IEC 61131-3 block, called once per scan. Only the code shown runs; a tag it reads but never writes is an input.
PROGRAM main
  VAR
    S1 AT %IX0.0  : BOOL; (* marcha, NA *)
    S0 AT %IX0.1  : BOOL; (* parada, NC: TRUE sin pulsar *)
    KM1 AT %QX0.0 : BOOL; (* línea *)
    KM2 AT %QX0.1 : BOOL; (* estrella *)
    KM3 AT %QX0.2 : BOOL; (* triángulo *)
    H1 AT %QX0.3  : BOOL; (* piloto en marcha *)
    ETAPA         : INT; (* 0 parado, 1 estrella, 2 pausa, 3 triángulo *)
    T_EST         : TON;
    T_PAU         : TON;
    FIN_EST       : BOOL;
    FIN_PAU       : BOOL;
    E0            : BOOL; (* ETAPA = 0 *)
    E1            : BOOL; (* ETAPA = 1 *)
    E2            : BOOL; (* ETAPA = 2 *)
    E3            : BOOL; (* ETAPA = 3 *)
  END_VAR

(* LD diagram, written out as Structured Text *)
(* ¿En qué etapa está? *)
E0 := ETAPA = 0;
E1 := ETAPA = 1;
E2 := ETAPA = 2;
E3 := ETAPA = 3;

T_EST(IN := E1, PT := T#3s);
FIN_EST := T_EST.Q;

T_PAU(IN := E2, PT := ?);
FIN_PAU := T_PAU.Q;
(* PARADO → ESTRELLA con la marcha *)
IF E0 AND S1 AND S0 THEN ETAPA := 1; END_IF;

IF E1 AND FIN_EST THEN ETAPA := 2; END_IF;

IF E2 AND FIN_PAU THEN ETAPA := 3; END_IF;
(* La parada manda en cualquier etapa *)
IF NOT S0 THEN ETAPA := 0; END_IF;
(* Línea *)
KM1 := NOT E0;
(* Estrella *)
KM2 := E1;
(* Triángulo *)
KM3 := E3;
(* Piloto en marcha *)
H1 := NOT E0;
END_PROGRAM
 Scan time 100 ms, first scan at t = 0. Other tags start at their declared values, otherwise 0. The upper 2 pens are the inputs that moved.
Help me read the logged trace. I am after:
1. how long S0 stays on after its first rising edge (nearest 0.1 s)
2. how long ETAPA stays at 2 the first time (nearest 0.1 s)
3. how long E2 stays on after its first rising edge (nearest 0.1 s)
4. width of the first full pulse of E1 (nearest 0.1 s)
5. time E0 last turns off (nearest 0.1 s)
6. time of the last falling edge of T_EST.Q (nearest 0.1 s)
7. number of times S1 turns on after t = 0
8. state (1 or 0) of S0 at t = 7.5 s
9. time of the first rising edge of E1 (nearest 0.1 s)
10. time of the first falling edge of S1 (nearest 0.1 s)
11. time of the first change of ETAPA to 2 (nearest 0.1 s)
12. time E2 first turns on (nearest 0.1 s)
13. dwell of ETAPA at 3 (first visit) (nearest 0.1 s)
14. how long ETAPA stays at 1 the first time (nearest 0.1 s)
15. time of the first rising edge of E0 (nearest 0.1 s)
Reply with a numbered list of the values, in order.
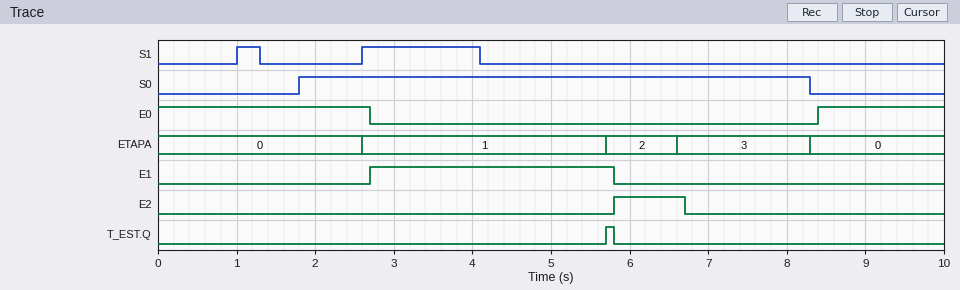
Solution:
1. 6.5 s
2. 0.9 s
3. 0.9 s
4. 3.1 s
5. 2.7 s
6. 5.8 s
7. 2
8. 1
9. 2.7 s
10. 1.3 s
11. 5.7 s
12. 5.8 s
13. 1.7 s
14. 3.1 s
15. 8.4 s
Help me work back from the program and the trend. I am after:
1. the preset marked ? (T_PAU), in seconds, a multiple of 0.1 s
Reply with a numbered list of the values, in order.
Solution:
1. 0.8 s
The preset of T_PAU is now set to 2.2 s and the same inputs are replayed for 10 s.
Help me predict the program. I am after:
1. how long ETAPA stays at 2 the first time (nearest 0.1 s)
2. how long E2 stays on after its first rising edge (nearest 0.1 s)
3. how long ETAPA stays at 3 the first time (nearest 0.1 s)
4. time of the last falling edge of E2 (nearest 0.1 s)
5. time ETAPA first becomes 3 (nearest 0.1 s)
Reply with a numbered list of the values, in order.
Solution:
1. 2.3 s
2. 2.3 s
3. 0.3 s
4. 8.1 s
5. 8.0 s
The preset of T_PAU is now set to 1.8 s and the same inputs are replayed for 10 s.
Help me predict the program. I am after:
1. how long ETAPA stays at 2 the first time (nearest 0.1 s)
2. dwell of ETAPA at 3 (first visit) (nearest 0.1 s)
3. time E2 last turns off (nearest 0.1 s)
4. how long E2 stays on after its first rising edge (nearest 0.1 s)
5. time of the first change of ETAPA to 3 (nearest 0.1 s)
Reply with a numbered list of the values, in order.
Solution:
1. 1.9 s
2. 0.7 s
3. 7.7 s
4. 1.9 s
5. 7.6 s
